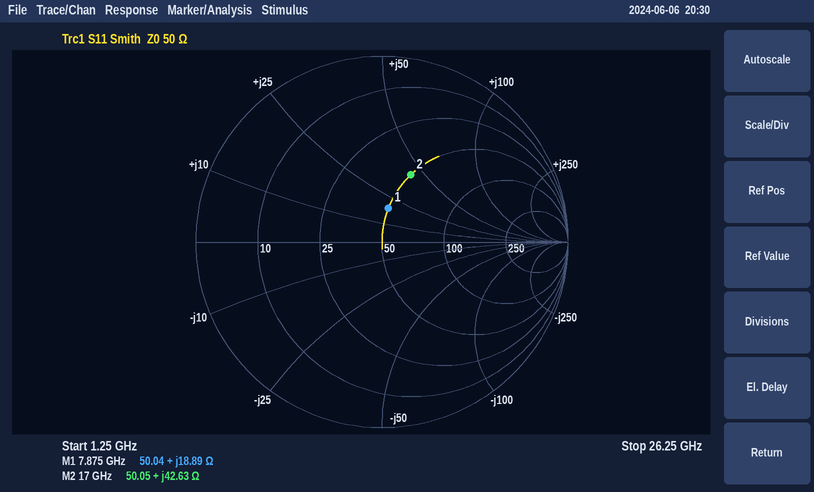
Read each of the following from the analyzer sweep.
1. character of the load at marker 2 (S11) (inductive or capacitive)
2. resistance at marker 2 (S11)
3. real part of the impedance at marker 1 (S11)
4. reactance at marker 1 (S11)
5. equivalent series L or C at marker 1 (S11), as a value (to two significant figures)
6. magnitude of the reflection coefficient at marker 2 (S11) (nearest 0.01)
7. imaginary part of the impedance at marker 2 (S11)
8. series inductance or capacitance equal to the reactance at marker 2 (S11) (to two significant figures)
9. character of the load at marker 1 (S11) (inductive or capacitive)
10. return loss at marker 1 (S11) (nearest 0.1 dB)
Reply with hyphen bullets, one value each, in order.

- inductive
- 50.05 Ω
- 50.04 Ω
- +18.89 Ω
- 380 pH
- 0.39
- +42.63 Ω
- 400 pH
- inductive
- 14.6 dB
